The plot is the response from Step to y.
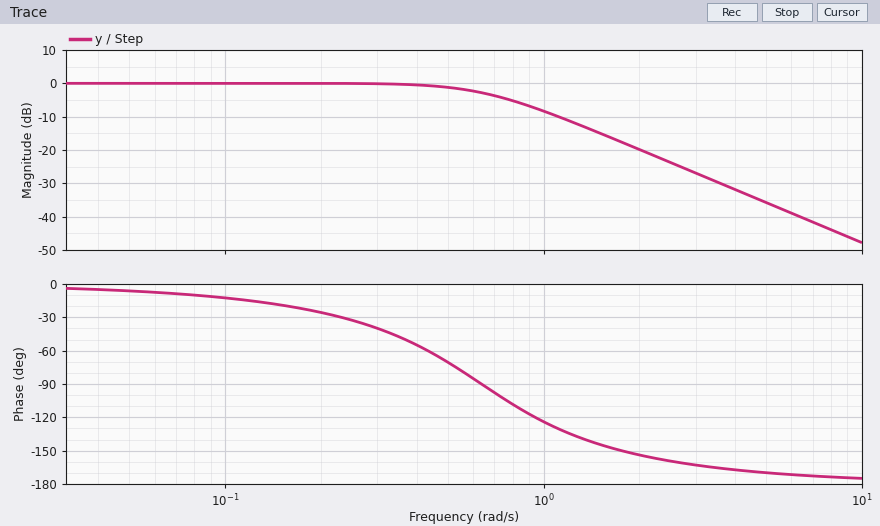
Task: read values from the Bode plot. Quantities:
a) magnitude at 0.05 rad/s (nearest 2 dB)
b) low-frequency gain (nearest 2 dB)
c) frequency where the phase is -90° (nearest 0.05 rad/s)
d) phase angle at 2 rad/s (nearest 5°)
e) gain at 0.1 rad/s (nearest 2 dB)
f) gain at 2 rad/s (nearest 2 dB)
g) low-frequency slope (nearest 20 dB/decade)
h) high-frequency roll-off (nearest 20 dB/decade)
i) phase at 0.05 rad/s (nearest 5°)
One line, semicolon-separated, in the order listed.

0 dB; 0 dB; 0.65 rad/s; -155°; 0 dB; -20 dB; 0 dB/decade; -40 dB/decade; -5°
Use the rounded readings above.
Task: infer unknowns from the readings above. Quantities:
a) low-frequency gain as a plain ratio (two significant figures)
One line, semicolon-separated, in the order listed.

1.0
